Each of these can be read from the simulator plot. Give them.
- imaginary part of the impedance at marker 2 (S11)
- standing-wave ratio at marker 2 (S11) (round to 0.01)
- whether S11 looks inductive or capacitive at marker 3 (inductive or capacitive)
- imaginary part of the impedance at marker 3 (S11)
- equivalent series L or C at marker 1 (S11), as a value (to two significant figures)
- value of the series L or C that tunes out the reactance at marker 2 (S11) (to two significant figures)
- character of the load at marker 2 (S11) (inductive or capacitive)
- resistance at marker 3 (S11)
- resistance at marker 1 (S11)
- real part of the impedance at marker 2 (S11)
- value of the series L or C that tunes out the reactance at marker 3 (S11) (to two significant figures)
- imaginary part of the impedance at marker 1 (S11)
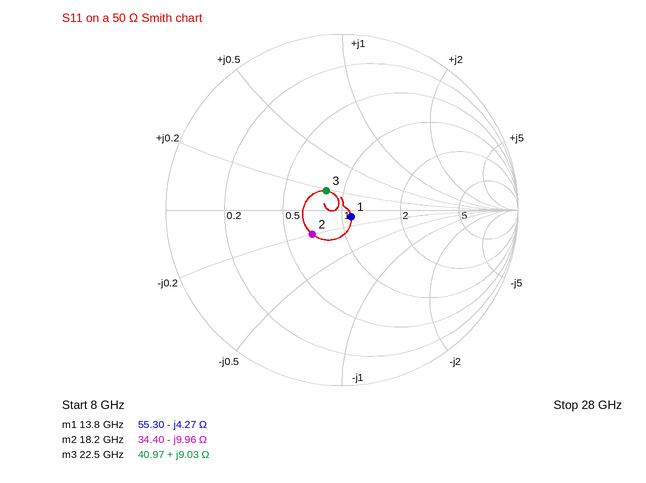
-9.96 Ω
1.56
inductive
+9.03 Ω
2.7 pF
87 pH
capacitive
40.97 Ω
55.30 Ω
34.40 Ω
780 fF
-4.27 Ω
